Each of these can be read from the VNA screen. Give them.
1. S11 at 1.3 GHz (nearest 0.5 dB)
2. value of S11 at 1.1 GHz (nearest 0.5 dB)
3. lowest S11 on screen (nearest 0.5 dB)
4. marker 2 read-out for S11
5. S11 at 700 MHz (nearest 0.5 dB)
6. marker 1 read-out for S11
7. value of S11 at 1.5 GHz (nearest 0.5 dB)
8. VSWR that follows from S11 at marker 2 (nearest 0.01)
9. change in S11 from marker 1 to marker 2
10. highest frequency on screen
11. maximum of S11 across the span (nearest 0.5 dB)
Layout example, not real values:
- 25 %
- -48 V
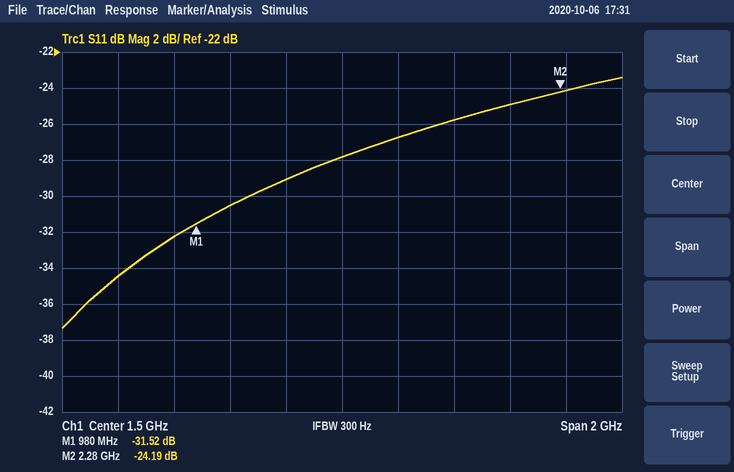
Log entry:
- -29.0 dB
- -30.5 dB
- -37.5 dB
- -24.19 dB
- -34.5 dB
- -31.52 dB
- -28.0 dB
- 1.13
- 7.33 dB
- 2.5 GHz
- -23.5 dB
